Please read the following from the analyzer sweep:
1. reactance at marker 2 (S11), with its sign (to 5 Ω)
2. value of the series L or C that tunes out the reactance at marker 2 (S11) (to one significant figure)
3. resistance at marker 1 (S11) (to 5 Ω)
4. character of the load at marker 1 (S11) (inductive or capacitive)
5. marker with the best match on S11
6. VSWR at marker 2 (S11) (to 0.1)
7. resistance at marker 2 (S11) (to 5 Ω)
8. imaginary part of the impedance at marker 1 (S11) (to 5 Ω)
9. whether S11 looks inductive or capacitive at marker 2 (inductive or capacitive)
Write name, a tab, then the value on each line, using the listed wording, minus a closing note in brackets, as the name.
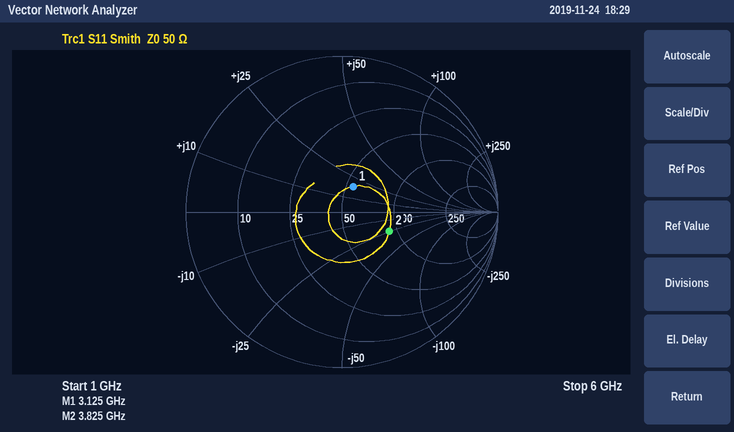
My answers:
reactance at marker 2 (S11), with its sign	-25 Ω
value of the series L or C that tunes out the reactance at marker 2 (S11)	1 nH
resistance at marker 1 (S11)	55 Ω
character of the load at marker 1 (S11)	inductive
marker with the best match on S11	marker 1
VSWR at marker 2 (S11)	2.0
resistance at marker 2 (S11)	90 Ω
imaginary part of the impedance at marker 1 (S11)	+20 Ω
whether S11 looks inductive or capacitive at marker 2	capacitive
